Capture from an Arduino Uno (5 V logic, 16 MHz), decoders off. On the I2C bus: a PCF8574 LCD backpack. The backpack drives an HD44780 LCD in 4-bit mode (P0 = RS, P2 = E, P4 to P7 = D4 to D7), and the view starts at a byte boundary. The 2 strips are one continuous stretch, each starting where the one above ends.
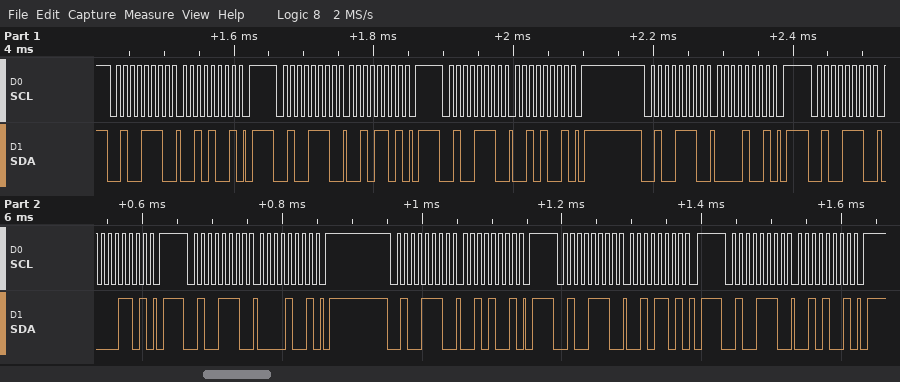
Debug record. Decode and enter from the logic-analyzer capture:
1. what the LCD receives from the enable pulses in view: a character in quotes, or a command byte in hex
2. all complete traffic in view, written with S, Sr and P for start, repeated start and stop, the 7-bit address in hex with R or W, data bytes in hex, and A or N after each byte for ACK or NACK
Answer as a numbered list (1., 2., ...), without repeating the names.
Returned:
1. ' '
2. S 27W A 29 A P S 27W A 2D A P S 27W A 29 A P S 27W A 09 A P S 27W A 0D A P S 27W A 09 A P S 27W A 29 A P S 27W A 2D A P S 27W A 29 A P
